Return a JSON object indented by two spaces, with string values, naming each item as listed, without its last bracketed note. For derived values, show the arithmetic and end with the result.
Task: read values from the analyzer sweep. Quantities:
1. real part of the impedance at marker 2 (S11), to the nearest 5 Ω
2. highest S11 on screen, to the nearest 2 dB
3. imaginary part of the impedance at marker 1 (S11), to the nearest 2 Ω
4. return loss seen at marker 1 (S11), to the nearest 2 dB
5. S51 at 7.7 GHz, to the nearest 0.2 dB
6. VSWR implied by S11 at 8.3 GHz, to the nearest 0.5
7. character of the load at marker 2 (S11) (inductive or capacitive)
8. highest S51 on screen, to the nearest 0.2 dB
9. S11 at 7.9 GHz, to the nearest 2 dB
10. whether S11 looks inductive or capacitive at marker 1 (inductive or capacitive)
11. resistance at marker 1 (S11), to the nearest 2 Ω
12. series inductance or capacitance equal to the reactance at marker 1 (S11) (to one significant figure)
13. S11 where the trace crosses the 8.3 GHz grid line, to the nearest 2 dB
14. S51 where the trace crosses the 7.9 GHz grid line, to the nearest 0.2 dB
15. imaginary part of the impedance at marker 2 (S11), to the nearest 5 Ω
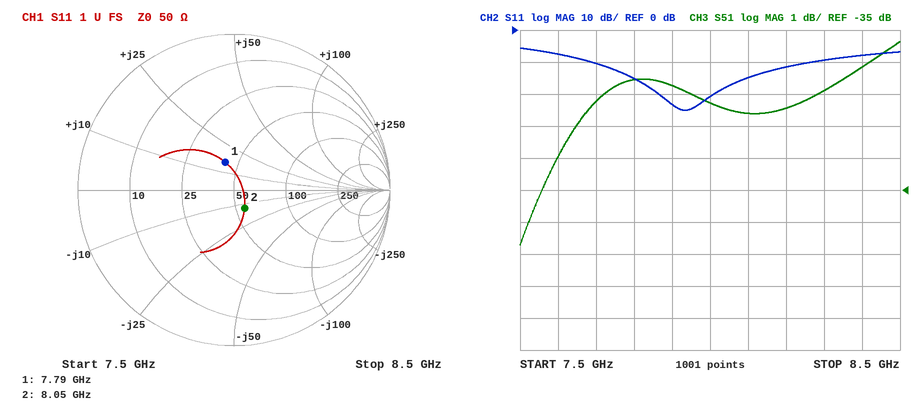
{
  "real part of the impedance at marker 2 (S11), to the nearest 5 Ω": "55 Ω",
  "highest S11 on screen, to the nearest 2 dB": "-6 dB",
  "imaginary part of the impedance at marker 1 (S11), to the nearest 2 Ω": "+16 Ω",
  "return loss seen at marker 1 (S11), to the nearest 2 dB": "14 dB",
  "S51 at 7.7 GHz, to the nearest 0.2 dB": "-32.2 dB",
  "VSWR implied by S11 at 8.3 GHz, to the nearest 0.5": "|Γ| = 10^(-10/20) = 0.3162; VSWR = (1 + 0.3162)/(1 − 0.3162) ≈ 1.92, so 2.0 to the nearest 0.5",
  "character of the load at marker 2 (S11)": "capacitive",
  "highest S51 on screen, to the nearest 0.2 dB": "-30.4 dB",
  "S11 at 7.9 GHz, to the nearest 2 dB": "-24 dB",
  "whether S11 looks inductive or capacitive at marker 1": "inductive",
  "resistance at marker 1 (S11), to the nearest 2 Ω": "42 Ω",
  "series inductance or capacitance equal to the reactance at marker 1 (S11)": "L = 16 Ω/(2π × 7.79 GHz) ≈ 327 pH, so 300 pH to one significant figure",
  "S11 where the trace crosses the 8.3 GHz grid line, to the nearest 2 dB": "-10 dB",
  "S51 where the trace crosses the 7.9 GHz grid line, to the nearest 0.2 dB": "-31.8 dB",
  "imaginary part of the impedance at marker 2 (S11), to the nearest 5 Ω": "-15 Ω"
}
